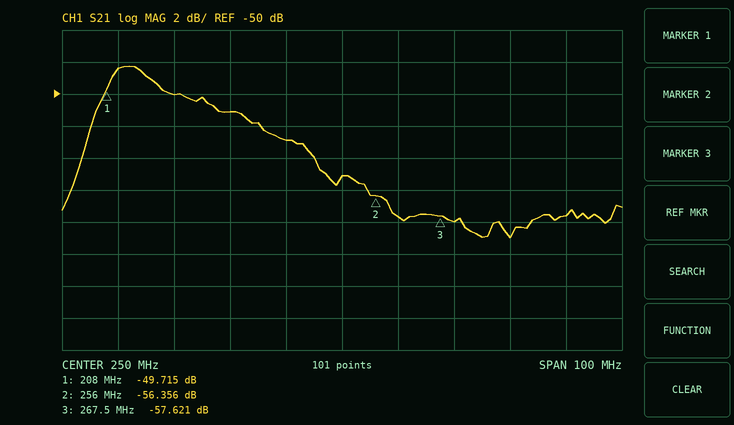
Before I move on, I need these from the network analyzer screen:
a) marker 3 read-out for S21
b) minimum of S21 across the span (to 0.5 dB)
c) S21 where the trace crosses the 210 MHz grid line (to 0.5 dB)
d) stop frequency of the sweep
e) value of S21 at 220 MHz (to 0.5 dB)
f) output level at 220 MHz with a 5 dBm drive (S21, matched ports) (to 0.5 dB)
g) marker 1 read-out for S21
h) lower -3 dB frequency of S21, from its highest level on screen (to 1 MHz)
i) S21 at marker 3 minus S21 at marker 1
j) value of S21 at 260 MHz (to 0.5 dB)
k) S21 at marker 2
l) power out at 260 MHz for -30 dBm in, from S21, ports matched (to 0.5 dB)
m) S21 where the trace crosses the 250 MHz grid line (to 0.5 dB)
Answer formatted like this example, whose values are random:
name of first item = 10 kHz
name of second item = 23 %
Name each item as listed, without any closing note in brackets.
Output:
marker 3 read-out for S21 = -57.621 dB
minimum of S21 across the span = -59.0 dB
S21 where the trace crosses the 210 MHz grid line = -48.5 dB
stop frequency of the sweep = 300 MHz
value of S21 at 220 MHz = -50.0 dB
output level at 220 MHz with a 5 dBm drive (S21, matched ports) = -45.0 dBm
marker 1 read-out for S21 = -49.715 dB
lower -3 dB frequency of S21, from its highest level on screen = 206 MHz
S21 at marker 3 minus S21 at marker 1 = -7.906 dB
value of S21 at 260 MHz = -57.5 dB
S21 at marker 2 = -56.356 dB
power out at 260 MHz for -30 dBm in, from S21, ports matched = -87.5 dBm
S21 where the trace crosses the 250 MHz grid line = -55.0 dB
